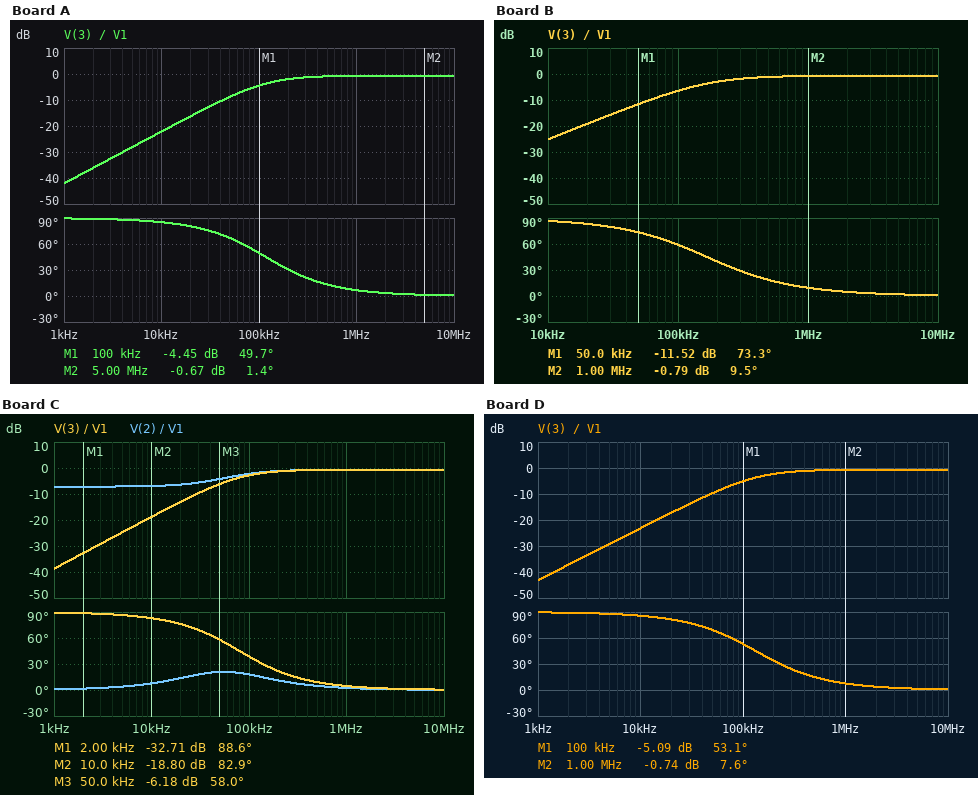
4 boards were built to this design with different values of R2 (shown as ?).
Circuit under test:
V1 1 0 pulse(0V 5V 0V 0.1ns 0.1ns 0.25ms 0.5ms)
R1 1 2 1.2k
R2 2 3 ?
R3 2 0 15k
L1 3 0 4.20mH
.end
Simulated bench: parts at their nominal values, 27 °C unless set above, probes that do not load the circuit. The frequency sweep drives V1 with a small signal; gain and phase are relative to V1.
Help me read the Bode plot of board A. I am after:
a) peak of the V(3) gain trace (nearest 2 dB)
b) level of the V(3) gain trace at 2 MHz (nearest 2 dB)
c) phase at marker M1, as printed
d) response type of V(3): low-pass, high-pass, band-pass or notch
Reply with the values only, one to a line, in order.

0 dB
0 dB
49.7 deg
high-pass
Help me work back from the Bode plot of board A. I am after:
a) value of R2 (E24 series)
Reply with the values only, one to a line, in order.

2 kΩ
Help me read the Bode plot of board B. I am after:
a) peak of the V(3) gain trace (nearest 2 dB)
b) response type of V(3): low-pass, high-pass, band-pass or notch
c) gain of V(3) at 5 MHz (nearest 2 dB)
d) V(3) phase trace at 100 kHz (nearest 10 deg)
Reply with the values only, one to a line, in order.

0 dB
high-pass
0 dB
60 deg
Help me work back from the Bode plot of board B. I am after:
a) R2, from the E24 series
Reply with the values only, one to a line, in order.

3.3 kΩ
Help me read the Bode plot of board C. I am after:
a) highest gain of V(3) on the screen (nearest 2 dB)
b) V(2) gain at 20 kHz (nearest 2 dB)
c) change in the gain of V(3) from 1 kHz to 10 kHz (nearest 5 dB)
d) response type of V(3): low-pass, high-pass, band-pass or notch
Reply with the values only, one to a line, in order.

0 dB
-6 dB
20 dB
high-pass
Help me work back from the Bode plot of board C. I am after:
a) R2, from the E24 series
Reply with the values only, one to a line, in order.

1 kΩ
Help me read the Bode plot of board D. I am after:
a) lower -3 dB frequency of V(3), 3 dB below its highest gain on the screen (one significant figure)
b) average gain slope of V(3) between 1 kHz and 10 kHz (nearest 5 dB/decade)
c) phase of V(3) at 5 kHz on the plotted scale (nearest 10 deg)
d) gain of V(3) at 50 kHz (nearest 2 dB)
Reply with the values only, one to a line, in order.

100 kHz
20 dB/decade
90 deg
-10 dB
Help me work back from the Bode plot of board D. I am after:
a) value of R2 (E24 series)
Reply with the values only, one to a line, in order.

2.4 kΩ
